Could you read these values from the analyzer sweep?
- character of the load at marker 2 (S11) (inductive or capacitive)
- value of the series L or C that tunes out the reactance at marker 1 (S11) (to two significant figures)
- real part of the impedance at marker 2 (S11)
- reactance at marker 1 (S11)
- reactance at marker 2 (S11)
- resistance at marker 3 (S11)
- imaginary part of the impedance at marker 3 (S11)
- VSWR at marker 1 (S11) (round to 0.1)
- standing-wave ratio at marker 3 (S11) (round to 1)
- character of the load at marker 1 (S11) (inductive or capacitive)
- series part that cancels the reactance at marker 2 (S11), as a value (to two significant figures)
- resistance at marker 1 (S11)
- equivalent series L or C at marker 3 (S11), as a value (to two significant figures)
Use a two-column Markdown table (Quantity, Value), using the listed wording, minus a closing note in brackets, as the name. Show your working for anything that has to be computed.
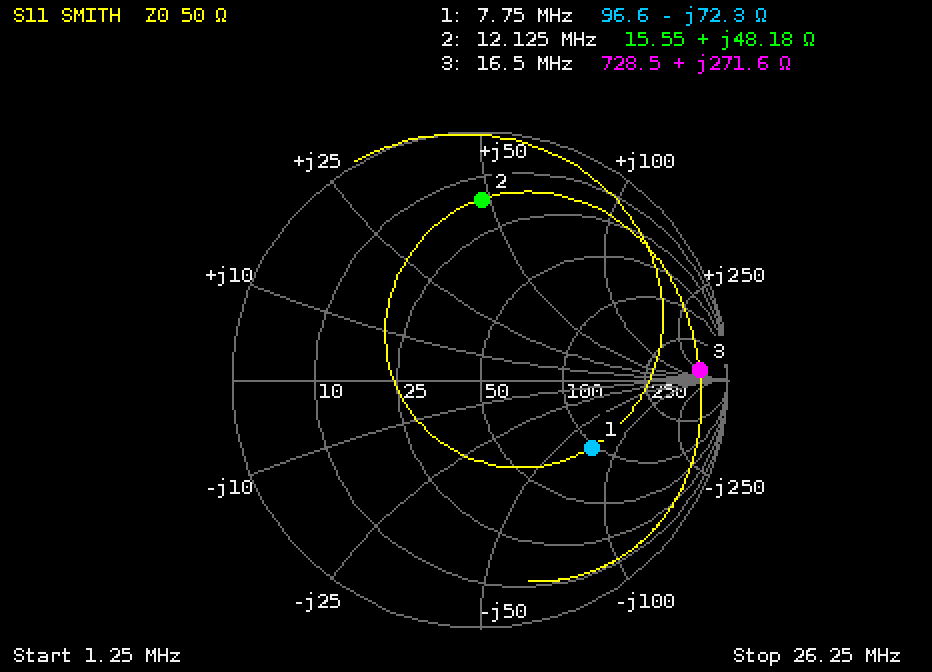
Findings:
| Quantity | Value |
|---|---|
| character of the load at marker 2 (S11) | inductive |
| value of the series L or C that tunes out the reactance at marker 1 (S11) | L = 72.3 Ω/(2π × 7.75 MHz) ≈ 1.5 µH |
| real part of the impedance at marker 2 | 15.55 Ω |
| reactance at marker 1 | -72.3 Ω |
| reactance at marker 2 | +48.18 Ω |
| resistance at marker 3 | 728.5 Ω |
| imaginary part of the impedance at marker 3 | +271.6 Ω |
| VSWR at marker 1 (S11) | 3.2 |
| standing-wave ratio at marker 3 (S11) | 17 |
| character of the load at marker 1 (S11) | capacitive |
| series part that cancels the reactance at marker 2 (S11), as a value | C = 1/(2π × 12.125 MHz × 48.18 Ω) ≈ 272 pF, so 270 pF to two significant figures |
| resistance at marker 1 | 96.6 Ω |
| equivalent series L or C at marker 3 (S11), as a value | L = 271.6 Ω/(2π × 16.5 MHz) ≈ 2.6 µH |
